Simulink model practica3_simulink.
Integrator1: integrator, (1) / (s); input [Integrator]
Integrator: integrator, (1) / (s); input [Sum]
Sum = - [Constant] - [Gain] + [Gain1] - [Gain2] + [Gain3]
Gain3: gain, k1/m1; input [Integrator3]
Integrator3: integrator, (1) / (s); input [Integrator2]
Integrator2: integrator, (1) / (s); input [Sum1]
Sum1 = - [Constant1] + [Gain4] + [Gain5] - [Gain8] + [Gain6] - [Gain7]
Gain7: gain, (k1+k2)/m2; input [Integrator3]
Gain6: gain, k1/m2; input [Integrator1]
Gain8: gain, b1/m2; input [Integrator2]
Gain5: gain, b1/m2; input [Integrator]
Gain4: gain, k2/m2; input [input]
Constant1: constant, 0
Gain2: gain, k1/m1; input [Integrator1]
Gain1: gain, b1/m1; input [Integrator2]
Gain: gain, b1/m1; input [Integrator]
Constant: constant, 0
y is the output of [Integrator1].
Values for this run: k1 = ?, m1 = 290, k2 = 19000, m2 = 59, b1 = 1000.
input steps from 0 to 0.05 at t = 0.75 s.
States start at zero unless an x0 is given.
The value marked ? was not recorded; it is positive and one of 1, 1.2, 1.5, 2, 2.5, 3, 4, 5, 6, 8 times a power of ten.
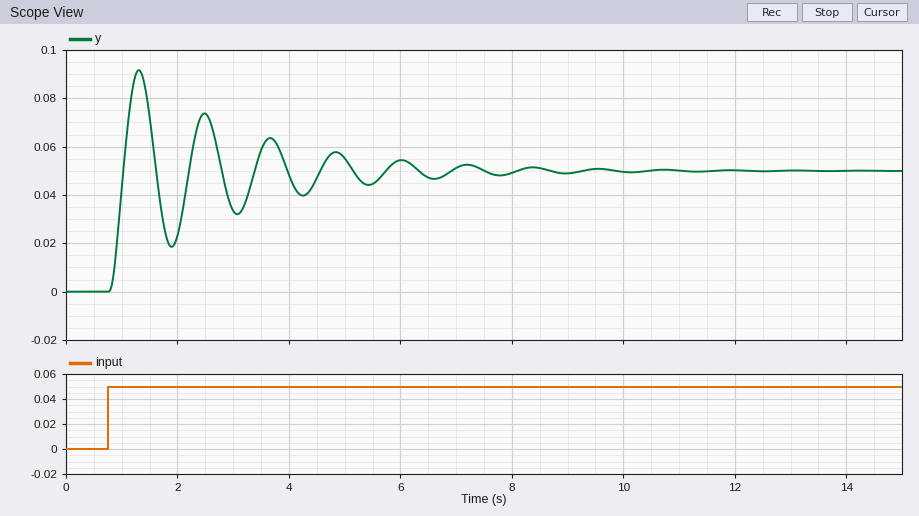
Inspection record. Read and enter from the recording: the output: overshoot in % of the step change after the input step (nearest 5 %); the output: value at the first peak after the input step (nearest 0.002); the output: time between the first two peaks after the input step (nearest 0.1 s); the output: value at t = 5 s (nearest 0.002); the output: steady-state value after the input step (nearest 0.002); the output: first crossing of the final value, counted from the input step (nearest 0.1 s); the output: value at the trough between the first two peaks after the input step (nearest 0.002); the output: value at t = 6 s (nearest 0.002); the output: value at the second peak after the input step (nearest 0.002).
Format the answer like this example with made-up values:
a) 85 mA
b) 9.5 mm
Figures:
a) 85 %
b) 0.092
c) 1.2 s
d) 0.056
e) 0.050
f) 0.3 s
g) 0.018
h) 0.054
i) 0.074
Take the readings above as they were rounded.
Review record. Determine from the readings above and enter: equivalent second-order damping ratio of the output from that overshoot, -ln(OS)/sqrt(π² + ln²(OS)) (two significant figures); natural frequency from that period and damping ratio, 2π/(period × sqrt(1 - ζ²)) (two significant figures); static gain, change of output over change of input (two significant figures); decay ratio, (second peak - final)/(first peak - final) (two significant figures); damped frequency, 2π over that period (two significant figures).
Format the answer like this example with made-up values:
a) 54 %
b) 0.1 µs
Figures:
a) 0.052
b) 5.2 rad/s
c) 1.0
d) 0.57
e) 5.2 rad/s
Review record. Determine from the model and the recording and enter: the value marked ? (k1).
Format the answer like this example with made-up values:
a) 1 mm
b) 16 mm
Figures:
a) 15000
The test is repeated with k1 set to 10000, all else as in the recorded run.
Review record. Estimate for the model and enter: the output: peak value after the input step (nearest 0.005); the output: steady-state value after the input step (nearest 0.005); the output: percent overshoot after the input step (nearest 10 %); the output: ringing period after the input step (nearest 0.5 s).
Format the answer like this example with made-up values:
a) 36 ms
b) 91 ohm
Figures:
a) 0.085
b) 0.050
c) 70 %
d) 1.5 s
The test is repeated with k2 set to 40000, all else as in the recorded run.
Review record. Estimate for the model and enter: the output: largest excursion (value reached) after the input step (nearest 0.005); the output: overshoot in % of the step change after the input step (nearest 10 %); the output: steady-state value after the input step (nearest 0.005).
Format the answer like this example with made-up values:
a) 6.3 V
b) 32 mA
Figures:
a) 0.085
b) 70 %
c) 0.050
